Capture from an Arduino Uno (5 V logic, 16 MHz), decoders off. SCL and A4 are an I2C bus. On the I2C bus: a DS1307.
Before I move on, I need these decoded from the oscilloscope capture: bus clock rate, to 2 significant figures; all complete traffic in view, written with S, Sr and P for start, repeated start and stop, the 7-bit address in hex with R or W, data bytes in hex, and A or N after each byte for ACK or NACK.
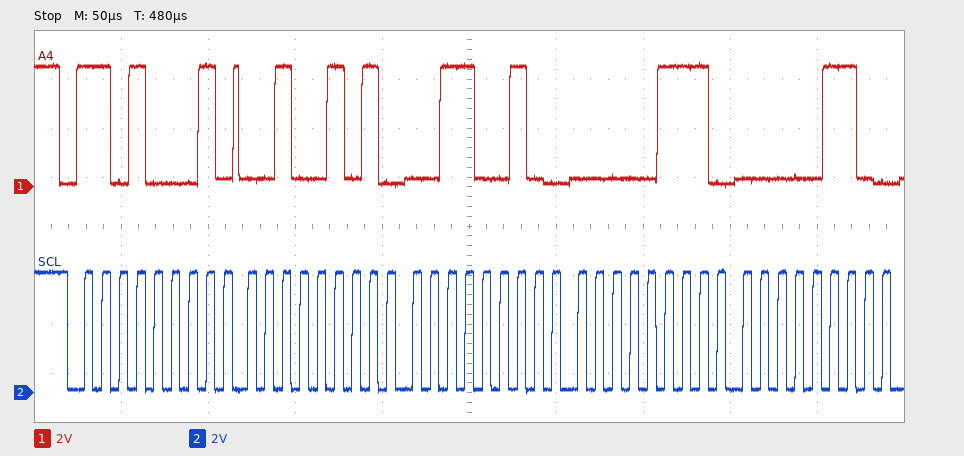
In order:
100 kHz
S 68R A 25 A 32 A 07 A 06 A
